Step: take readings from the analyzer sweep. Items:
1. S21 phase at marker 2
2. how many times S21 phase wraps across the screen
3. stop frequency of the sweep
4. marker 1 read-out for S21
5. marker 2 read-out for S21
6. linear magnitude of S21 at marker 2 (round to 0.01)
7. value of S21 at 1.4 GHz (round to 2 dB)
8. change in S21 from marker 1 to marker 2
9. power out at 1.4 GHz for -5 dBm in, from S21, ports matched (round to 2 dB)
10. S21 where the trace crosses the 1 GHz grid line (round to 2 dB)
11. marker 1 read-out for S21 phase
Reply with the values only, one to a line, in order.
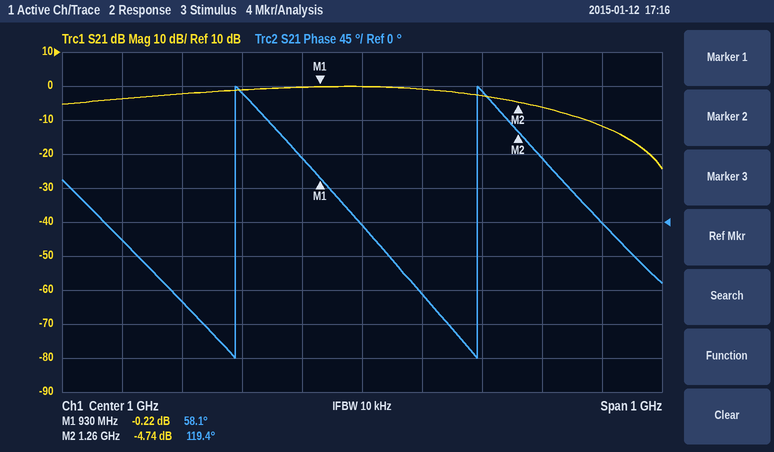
119.4°
2
1.5 GHz
-0.22 dB
-4.74 dB
0.58
-12 dB
-4.52 dB
-16 dBm
0 dB
58.1°
